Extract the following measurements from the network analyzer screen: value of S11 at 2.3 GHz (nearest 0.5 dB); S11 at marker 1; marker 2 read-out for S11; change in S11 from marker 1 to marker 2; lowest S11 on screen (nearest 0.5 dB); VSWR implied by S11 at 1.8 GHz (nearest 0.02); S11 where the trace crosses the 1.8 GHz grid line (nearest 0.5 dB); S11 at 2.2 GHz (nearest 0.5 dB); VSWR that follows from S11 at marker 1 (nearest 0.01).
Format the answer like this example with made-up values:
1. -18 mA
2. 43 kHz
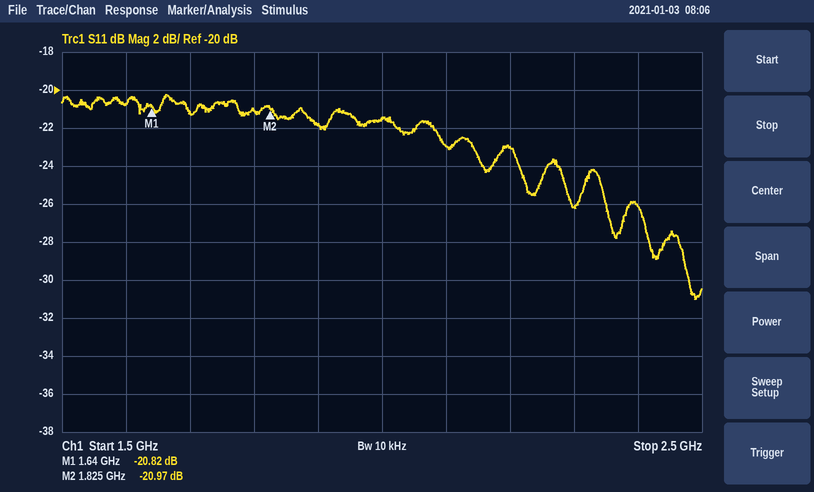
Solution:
1. -26.0 dB
2. -20.82 dB
3. -20.97 dB
4. -0.15 dB
5. -31.0 dB
6. 1.20
7. -21.0 dB
8. -23.0 dB
9. 1.20
